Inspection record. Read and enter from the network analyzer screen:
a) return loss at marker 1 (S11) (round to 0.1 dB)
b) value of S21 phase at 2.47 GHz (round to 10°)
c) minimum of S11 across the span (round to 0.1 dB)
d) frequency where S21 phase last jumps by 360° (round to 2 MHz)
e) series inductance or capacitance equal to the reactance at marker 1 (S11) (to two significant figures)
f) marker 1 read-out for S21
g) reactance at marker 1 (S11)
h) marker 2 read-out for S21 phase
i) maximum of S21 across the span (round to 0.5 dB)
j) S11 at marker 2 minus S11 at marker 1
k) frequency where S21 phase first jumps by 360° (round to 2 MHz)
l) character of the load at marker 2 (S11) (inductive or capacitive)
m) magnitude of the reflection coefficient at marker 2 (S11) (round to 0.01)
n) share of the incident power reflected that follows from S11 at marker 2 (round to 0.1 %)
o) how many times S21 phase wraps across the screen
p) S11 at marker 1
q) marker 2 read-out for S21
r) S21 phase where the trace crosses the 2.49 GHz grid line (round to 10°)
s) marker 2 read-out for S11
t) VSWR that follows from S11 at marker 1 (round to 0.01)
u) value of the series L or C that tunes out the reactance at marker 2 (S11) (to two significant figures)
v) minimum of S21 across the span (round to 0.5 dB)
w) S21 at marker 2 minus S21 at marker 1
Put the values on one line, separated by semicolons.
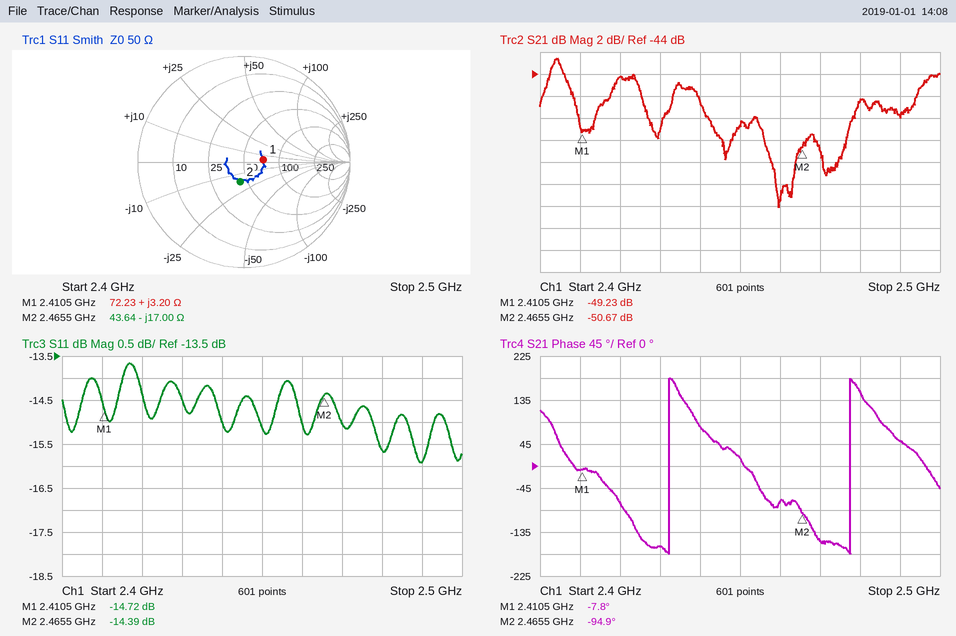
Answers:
14.7 dB; -150°; -15.9 dB; 2.478 GHz; 210 pH; -49.23 dB; +3.20 Ω; -94.9°; -42.5 dB; 0.33 dB; 2.432 GHz; capacitive; 0.19; 3.6 %; 2; -14.72 dB; -50.67 dB; 50°; -14.39 dB; 1.45; 1.1 nH; -56.0 dB; -1.44 dB
